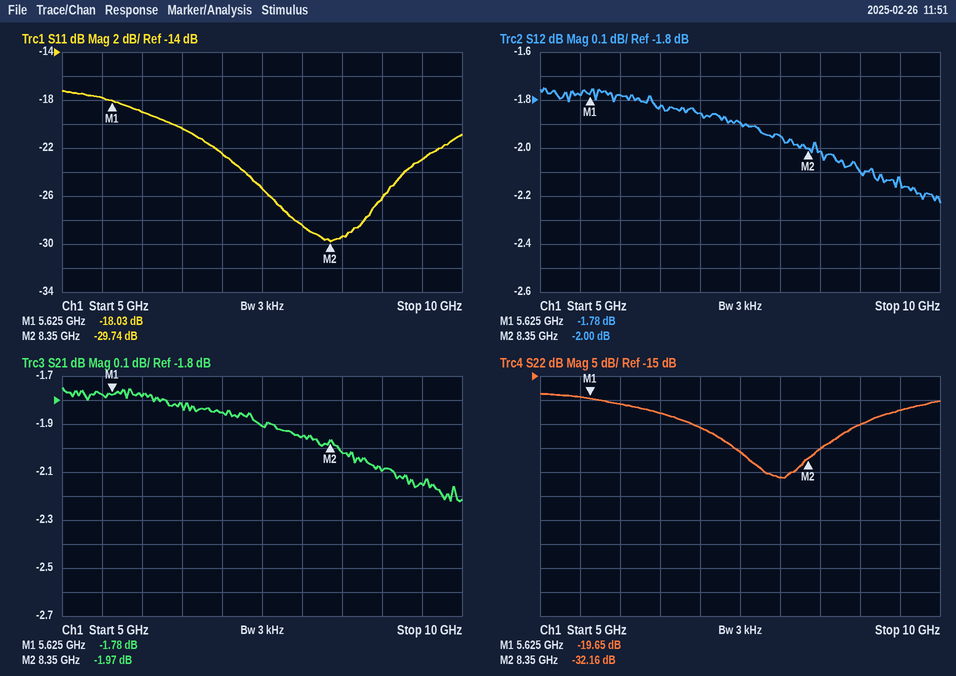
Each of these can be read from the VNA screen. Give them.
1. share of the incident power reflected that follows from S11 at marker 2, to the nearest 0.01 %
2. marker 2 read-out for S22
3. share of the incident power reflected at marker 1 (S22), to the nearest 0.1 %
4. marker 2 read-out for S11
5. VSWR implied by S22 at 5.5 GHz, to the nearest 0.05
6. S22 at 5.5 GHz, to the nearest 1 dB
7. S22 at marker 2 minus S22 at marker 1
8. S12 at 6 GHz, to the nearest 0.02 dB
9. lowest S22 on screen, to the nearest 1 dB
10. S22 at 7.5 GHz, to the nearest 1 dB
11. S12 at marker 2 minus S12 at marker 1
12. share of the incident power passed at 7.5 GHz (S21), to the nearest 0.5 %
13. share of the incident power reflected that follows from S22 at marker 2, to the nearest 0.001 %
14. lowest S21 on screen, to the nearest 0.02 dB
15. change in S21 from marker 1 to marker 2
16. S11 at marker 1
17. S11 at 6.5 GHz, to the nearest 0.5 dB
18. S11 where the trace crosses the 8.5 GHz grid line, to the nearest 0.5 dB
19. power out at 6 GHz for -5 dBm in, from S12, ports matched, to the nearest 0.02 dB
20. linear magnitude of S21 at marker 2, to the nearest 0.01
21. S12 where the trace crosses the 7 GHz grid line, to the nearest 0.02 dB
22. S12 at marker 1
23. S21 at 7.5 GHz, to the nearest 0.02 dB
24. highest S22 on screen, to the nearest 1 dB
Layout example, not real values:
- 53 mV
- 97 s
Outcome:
- 0.11 %
- -32.16 dB
- 1.1 %
- -29.74 dB
- 1.25
- -19 dB
- -12.51 dB
- -1.78 dB
- -36 dB
- -31 dB
- -0.22 dB
- 64.5 %
- 0.061 %
- -2.22 dB
- -0.19 dB
- -18.03 dB
- -20.5 dB
- -29.5 dB
- -6.78 dBm
- 0.80
- -1.86 dB
- -1.78 dB
- -1.90 dB
- -19 dB
